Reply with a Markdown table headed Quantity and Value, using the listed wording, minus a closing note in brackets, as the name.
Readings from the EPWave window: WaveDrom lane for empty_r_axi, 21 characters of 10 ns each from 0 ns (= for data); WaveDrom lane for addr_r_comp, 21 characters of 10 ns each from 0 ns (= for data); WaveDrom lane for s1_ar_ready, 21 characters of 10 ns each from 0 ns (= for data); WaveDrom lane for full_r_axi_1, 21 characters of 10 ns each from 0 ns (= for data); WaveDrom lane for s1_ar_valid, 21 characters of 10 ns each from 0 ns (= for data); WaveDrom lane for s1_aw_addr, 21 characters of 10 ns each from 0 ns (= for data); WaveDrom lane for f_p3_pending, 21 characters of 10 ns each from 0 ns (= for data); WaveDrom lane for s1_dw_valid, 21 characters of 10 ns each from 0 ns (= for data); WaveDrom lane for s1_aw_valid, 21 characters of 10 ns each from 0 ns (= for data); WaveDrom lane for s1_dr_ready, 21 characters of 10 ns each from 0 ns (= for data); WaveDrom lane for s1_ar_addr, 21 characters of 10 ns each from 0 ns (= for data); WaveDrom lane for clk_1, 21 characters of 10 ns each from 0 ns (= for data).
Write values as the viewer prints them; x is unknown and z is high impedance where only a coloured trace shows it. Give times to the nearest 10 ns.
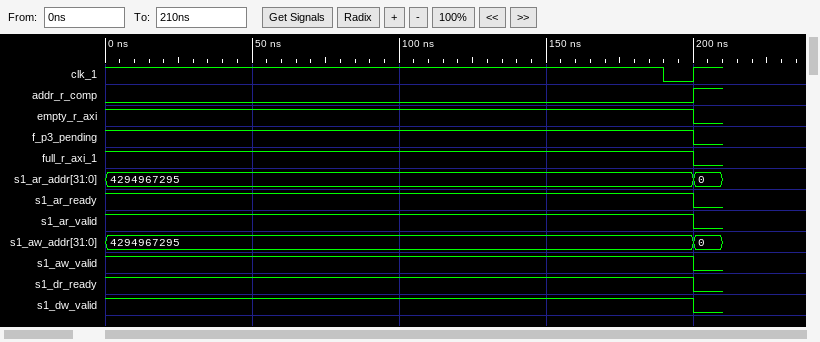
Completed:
| Quantity | Value |
|---|---|
| WaveDrom lane for empty_r_axi, 21 characters of 10 ns each from 0 ns | {name: 'empty_r_axi', wave: '1...................0'} |
| WaveDrom lane for addr_r_comp, 21 characters of 10 ns each from 0 ns | {name: 'addr_r_comp', wave: '0...................1'} |
| WaveDrom lane for s1_ar_ready, 21 characters of 10 ns each from 0 ns | {name: 's1_ar_ready', wave: '1...................0'} |
| WaveDrom lane for full_r_axi_1, 21 characters of 10 ns each from 0 ns | {name: 'full_r_axi_1', wave: '1...................0'} |
| WaveDrom lane for s1_ar_valid, 21 characters of 10 ns each from 0 ns | {name: 's1_ar_valid', wave: '1...................0'} |
| WaveDrom lane for s1_aw_addr, 21 characters of 10 ns each from 0 ns | {name: 's1_aw_addr', wave: '=...................=', data: '4294967295 0'} |
| WaveDrom lane for f_p3_pending, 21 characters of 10 ns each from 0 ns | {name: 'f_p3_pending', wave: '1...................0'} |
| WaveDrom lane for s1_dw_valid, 21 characters of 10 ns each from 0 ns | {name: 's1_dw_valid', wave: '1...................0'} |
| WaveDrom lane for s1_aw_valid, 21 characters of 10 ns each from 0 ns | {name: 's1_aw_valid', wave: '1...................0'} |
| WaveDrom lane for s1_dr_ready, 21 characters of 10 ns each from 0 ns | {name: 's1_dr_ready', wave: '1...................0'} |
| WaveDrom lane for s1_ar_addr, 21 characters of 10 ns each from 0 ns | {name: 's1_ar_addr', wave: '=...................=', data: '4294967295 0'} |
| WaveDrom lane for clk_1, 21 characters of 10 ns each from 0 ns | {name: 'clk_1', wave: '1..................01'} |
